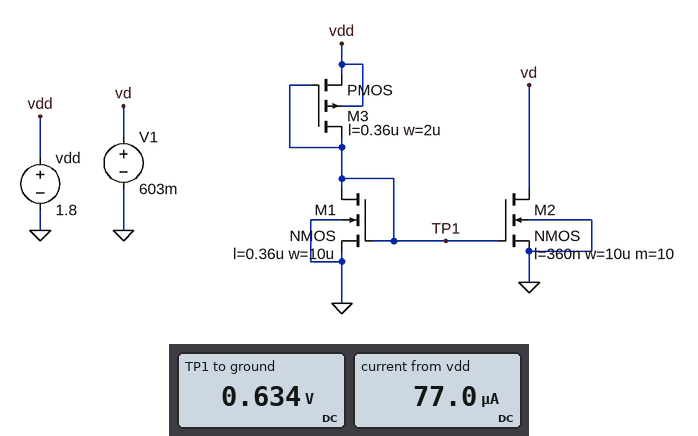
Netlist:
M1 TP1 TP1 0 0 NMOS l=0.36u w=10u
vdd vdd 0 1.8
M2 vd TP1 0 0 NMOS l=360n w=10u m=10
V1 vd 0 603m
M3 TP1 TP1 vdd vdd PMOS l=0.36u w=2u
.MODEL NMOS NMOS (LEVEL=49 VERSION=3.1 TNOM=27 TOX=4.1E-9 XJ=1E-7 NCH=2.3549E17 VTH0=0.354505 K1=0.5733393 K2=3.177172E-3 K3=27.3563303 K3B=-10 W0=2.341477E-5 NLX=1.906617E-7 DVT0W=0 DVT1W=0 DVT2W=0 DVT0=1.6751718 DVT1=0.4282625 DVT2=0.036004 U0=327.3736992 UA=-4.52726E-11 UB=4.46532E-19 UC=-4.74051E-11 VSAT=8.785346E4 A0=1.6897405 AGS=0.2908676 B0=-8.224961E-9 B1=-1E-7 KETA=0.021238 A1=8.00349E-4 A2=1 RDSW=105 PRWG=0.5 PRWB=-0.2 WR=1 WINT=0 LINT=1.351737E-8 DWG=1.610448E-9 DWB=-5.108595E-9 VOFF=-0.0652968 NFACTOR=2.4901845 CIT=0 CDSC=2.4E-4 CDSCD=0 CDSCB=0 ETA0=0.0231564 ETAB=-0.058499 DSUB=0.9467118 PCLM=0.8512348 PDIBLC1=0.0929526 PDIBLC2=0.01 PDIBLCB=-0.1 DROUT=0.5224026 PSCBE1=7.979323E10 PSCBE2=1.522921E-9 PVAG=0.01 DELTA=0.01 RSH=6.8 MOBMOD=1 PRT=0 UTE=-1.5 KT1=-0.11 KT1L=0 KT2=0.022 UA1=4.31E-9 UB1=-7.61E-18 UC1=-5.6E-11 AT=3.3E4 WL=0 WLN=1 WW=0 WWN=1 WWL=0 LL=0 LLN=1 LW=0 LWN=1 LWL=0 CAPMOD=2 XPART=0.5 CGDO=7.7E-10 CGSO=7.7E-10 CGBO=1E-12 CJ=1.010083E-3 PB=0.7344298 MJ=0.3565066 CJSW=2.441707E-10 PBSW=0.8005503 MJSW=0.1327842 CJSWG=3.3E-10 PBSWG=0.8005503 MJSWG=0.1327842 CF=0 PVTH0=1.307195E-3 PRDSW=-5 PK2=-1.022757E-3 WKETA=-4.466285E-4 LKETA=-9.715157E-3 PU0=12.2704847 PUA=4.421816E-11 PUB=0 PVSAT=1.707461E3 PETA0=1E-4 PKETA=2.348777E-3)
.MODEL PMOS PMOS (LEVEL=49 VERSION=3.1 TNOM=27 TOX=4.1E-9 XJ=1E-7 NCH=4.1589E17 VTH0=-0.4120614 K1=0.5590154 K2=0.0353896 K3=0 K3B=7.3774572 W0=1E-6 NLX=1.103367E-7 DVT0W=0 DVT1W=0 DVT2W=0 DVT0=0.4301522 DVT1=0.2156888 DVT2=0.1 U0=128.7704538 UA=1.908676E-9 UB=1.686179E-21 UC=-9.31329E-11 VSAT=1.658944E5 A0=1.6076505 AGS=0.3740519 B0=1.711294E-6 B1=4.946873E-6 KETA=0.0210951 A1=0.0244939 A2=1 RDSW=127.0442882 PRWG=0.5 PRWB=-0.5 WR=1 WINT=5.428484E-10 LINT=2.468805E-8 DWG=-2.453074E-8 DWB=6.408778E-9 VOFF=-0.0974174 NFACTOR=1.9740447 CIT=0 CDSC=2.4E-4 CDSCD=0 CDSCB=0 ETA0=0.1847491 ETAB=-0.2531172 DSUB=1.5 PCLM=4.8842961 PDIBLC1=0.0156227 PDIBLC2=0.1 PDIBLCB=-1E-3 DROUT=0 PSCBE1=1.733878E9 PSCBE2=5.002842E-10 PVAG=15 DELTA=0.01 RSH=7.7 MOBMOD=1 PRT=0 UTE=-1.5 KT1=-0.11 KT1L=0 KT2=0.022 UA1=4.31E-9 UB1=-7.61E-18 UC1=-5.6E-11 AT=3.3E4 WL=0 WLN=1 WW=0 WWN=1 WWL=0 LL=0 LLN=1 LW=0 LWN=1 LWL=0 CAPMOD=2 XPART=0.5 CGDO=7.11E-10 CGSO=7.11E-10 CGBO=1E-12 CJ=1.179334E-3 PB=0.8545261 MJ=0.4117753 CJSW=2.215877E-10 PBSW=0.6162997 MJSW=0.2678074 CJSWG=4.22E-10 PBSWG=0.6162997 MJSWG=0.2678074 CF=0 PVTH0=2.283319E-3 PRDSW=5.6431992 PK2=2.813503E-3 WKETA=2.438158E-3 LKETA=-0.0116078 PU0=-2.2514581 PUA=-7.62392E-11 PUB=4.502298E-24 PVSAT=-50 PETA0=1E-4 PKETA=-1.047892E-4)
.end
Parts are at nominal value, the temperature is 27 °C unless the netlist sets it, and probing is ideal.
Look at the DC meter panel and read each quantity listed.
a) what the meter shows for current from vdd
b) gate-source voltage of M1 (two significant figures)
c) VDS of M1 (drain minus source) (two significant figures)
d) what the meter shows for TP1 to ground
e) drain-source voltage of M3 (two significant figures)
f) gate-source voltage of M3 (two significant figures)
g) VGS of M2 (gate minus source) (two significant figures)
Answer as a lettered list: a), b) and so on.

a) 77.0 µA
b) 630 mV
c) 630 mV
d) 0.634 V
e) -1.2 V
f) -1.2 V
g) 630 mV
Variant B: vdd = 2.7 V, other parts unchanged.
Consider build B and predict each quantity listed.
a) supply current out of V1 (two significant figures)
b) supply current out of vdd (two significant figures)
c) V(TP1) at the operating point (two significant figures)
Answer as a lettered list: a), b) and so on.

a) 2.7 mA
b) 280 µA
c) 770 mV
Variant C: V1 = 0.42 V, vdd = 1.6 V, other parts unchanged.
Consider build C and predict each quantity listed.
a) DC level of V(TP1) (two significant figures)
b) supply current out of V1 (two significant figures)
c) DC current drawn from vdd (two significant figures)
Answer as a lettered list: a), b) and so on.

a) 600 mV
b) 460 µA
c) 47 µA
